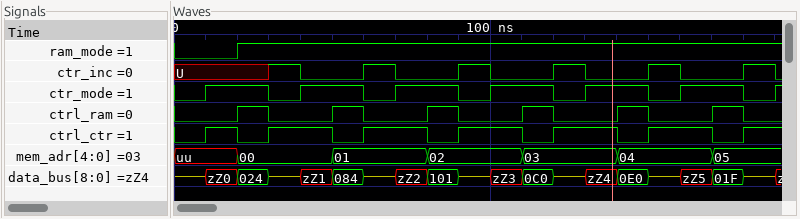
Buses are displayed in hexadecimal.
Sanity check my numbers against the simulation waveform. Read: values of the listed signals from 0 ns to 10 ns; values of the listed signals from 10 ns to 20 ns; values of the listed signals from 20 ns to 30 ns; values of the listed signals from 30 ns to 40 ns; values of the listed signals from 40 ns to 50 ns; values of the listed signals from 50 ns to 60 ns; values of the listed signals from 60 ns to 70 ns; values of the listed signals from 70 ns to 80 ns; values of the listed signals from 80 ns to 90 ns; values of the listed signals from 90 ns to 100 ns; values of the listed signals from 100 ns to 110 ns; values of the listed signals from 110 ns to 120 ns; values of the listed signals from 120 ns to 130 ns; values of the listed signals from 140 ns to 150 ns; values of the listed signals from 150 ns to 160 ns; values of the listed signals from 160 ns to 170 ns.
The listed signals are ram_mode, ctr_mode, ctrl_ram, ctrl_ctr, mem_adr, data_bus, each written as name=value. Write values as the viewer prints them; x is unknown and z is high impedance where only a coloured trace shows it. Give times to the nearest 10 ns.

ram_mode=0, ctr_mode=0, ctrl_ram=0, ctrl_ctr=0, mem_adr=uu, data_bus=z
ram_mode=0, ctr_mode=1, ctrl_ram=0, ctrl_ctr=1, mem_adr=uu, data_bus=zZ0
ram_mode=1, ctr_mode=1, ctrl_ram=1, ctrl_ctr=0, mem_adr=00, data_bus=024
ram_mode=1, ctr_mode=0, ctrl_ram=0, ctrl_ctr=1, mem_adr=00, data_bus=z
ram_mode=1, ctr_mode=1, ctrl_ram=0, ctrl_ctr=1, mem_adr=00, data_bus=zZ1
ram_mode=1, ctr_mode=1, ctrl_ram=1, ctrl_ctr=0, mem_adr=01, data_bus=084
ram_mode=1, ctr_mode=0, ctrl_ram=0, ctrl_ctr=1, mem_adr=01, data_bus=z
ram_mode=1, ctr_mode=1, ctrl_ram=0, ctrl_ctr=1, mem_adr=01, data_bus=zZ2
ram_mode=1, ctr_mode=1, ctrl_ram=1, ctrl_ctr=0, mem_adr=02, data_bus=101
ram_mode=1, ctr_mode=0, ctrl_ram=0, ctrl_ctr=1, mem_adr=02, data_bus=z
ram_mode=1, ctr_mode=1, ctrl_ram=0, ctrl_ctr=1, mem_adr=02, data_bus=zZ3
ram_mode=1, ctr_mode=1, ctrl_ram=1, ctrl_ctr=0, mem_adr=03, data_bus=0C0
ram_mode=1, ctr_mode=0, ctrl_ram=0, ctrl_ctr=1, mem_adr=03, data_bus=z
ram_mode=1, ctr_mode=1, ctrl_ram=1, ctrl_ctr=0, mem_adr=04, data_bus=0E0
ram_mode=1, ctr_mode=0, ctrl_ram=0, ctrl_ctr=1, mem_adr=04, data_bus=z
ram_mode=1, ctr_mode=1, ctrl_ram=0, ctrl_ctr=1, mem_adr=04, data_bus=zZ5
